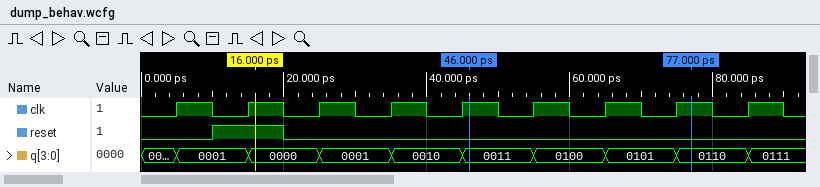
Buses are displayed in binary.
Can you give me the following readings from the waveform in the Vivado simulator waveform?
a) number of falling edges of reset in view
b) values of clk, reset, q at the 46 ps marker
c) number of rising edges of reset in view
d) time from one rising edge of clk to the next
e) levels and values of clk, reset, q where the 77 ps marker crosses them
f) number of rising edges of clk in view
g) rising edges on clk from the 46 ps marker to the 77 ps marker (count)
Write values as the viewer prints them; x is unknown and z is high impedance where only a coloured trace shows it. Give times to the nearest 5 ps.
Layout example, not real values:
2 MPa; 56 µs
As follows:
1; clk=1, reset=0, q=0011; 1; 10 ps; clk=1, reset=0, q=0110; 9; 3
